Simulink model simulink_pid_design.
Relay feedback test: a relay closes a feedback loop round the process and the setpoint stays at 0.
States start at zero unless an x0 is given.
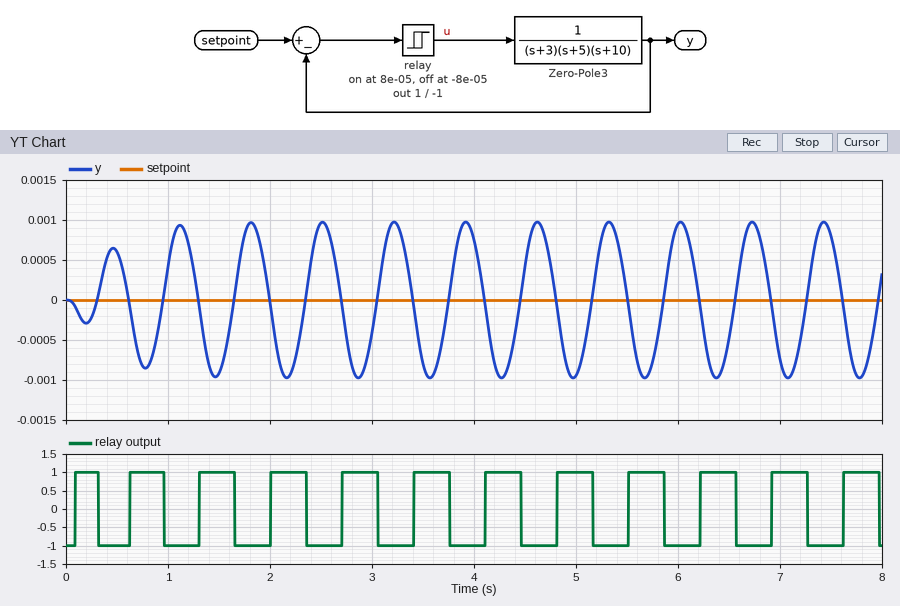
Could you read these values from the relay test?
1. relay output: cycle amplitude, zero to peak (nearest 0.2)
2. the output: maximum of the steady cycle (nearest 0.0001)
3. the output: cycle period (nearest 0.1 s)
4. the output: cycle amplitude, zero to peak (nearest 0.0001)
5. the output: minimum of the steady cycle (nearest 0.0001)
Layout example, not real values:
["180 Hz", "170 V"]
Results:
["1.0", "0.0010", "0.7 s", "0.0010", "-0.0010"]
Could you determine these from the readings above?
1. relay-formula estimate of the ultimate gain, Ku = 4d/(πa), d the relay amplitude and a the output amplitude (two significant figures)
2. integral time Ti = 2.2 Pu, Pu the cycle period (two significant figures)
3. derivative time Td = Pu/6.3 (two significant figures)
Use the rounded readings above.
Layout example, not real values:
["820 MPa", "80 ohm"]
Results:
["1300", "1.5 s", "0.11 s"]
